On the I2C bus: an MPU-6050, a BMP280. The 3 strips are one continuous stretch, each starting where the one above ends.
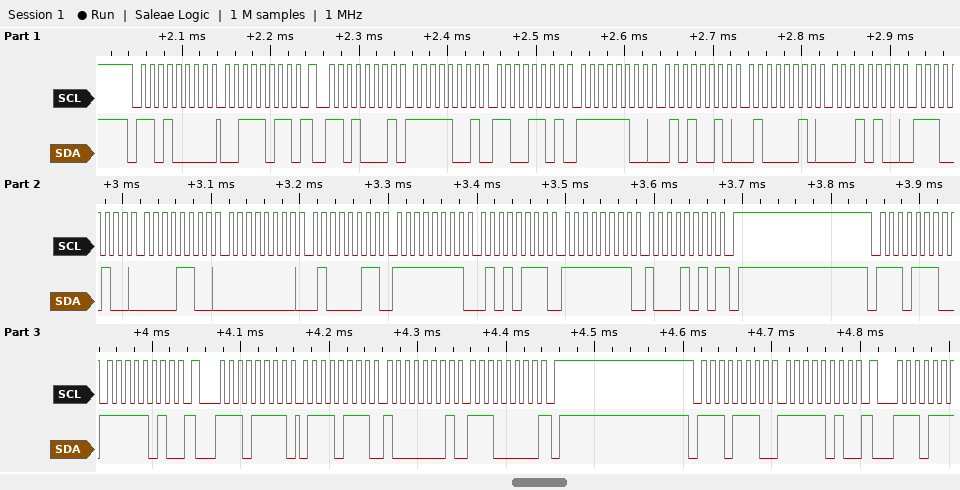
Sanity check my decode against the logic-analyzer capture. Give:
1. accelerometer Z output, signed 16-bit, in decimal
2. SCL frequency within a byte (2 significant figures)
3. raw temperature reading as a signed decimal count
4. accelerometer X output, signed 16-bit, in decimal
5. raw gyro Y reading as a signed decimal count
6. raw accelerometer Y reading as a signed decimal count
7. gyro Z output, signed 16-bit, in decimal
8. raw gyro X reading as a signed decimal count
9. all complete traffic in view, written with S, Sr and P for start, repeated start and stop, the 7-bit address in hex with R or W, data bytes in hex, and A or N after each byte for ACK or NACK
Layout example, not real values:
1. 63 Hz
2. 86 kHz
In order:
1. 16916
2. 100 kHz
3. -7156
4. -1587
5. -169
6. -942
7. -118
8. 67
9. S 68W A 3B A Sr 68R A F9 A CD A FC A 52 A 42 A 14 A E4 A 0C A 00 A 43 A FF A 57 A FF A 8A N P S 77W A FA A Sr 77R A 77 A 81 A E0 N P S 77W A FA A
